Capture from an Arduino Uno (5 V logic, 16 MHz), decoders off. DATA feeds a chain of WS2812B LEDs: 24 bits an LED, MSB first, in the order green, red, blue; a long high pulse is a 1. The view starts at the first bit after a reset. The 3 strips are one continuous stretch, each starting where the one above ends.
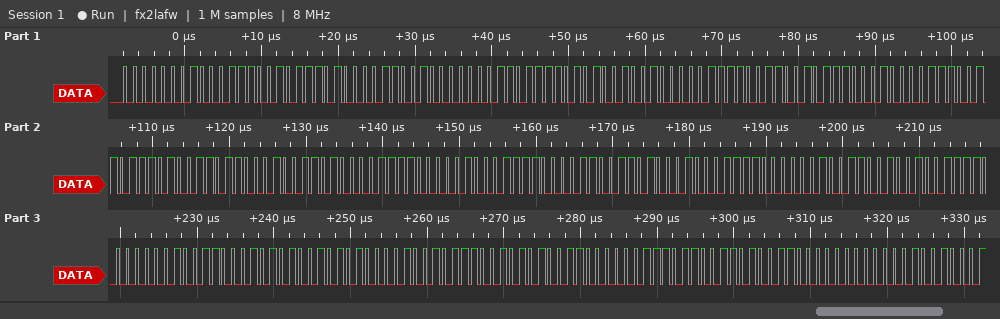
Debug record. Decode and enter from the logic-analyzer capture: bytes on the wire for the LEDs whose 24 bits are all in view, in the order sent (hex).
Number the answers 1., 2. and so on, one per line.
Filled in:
1. 01 1C BA 19 01 BD 49 07 99 71 0E 6E 9B 13 43 C1 1E 19 A2 3C 09 92 78 09 8A 95 09 72 A6 07 66 98 00
